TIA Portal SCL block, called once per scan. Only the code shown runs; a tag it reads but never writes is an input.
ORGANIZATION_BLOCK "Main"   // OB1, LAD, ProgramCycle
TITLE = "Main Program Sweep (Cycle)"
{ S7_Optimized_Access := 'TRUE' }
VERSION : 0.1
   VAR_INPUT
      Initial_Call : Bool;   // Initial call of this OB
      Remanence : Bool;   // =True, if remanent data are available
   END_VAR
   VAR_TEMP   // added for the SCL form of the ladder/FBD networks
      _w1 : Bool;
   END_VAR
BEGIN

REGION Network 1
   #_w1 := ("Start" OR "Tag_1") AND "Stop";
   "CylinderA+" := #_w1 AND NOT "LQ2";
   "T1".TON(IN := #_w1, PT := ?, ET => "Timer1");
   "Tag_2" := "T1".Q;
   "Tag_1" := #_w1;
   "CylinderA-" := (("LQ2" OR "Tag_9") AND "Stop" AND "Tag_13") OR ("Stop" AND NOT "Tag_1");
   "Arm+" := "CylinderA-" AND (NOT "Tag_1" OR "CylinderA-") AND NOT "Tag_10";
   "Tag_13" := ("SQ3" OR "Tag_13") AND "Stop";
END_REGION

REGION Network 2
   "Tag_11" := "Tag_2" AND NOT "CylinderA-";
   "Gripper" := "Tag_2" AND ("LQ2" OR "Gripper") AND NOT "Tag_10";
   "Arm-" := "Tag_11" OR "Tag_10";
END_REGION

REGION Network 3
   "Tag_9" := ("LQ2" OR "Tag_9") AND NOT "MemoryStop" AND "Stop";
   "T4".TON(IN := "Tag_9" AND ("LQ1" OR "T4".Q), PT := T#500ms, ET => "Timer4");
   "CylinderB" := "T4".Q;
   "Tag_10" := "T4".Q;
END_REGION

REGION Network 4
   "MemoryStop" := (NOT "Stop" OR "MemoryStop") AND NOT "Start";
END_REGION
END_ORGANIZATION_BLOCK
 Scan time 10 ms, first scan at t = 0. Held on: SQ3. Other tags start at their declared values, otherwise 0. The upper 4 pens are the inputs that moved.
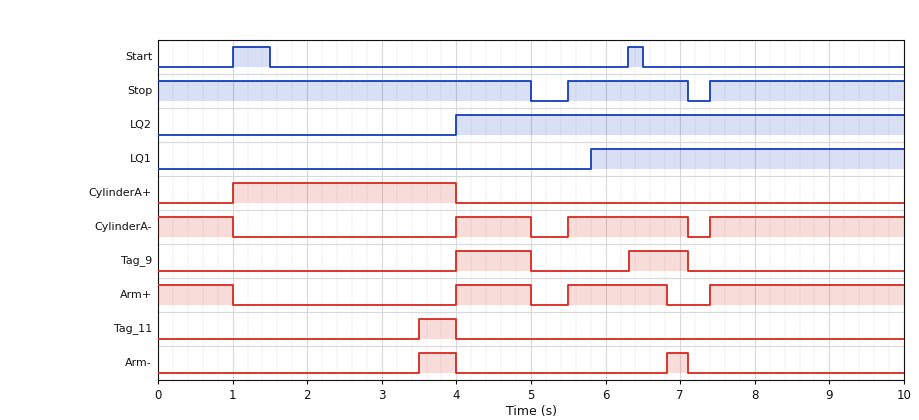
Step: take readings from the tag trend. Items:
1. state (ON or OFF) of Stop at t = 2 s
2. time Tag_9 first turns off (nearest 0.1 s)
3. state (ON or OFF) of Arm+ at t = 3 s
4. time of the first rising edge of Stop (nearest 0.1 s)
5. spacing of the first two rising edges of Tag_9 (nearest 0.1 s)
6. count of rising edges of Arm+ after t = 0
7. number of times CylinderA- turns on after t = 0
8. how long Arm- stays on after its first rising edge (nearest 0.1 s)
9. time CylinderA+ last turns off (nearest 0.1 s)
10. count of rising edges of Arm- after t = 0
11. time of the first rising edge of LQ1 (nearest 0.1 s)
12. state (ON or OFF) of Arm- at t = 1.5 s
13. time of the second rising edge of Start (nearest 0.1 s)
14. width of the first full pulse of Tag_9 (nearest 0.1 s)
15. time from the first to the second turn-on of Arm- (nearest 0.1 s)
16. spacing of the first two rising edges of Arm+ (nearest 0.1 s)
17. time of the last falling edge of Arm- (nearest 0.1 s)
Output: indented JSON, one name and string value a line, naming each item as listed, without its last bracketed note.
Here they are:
{
  "state (ON or OFF) of Stop at t = 2 s": "ON",
  "time Tag_9 first turns off": "5.0 s",
  "state (ON or OFF) of Arm+ at t = 3 s": "OFF",
  "time of the first rising edge of Stop": "5.5 s",
  "spacing of the first two rising edges of Tag_9": "2.3 s",
  "count of rising edges of Arm+ after t = 0": "3",
  "number of times CylinderA- turns on after t = 0": "3",
  "how long Arm- stays on after its first rising edge": "0.5 s",
  "time CylinderA+ last turns off": "4.0 s",
  "count of rising edges of Arm- after t = 0": "2",
  "time of the first rising edge of LQ1": "5.8 s",
  "state (ON or OFF) of Arm- at t = 1.5 s": "OFF",
  "time of the second rising edge of Start": "6.3 s",
  "width of the first full pulse of Tag_9": "1.0 s",
  "time from the first to the second turn-on of Arm-": "3.3 s",
  "spacing of the first two rising edges of Arm+": "1.5 s",
  "time of the last falling edge of Arm-": "7.1 s"
}
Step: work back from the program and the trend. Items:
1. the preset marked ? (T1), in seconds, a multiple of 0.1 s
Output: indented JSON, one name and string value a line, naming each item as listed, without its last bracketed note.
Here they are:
{
  "the preset marked ? (T1), in seconds, a multiple of 0.1 s": "2.5 s"
}
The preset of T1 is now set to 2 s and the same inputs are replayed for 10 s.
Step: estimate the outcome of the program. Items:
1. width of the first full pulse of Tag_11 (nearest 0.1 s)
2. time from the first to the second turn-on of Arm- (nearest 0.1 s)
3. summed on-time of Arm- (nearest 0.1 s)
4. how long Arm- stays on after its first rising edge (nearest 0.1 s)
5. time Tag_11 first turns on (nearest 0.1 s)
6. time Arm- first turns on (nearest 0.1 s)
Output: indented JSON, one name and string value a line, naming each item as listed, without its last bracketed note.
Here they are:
{
  "width of the first full pulse of Tag_11": "1.0 s",
  "time from the first to the second turn-on of Arm-": "3.8 s",
  "summed on-time of Arm-": "1.3 s",
  "how long Arm- stays on after its first rising edge": "1.0 s",
  "time Tag_11 first turns on": "3.0 s",
  "time Arm- first turns on": "3.0 s"
}
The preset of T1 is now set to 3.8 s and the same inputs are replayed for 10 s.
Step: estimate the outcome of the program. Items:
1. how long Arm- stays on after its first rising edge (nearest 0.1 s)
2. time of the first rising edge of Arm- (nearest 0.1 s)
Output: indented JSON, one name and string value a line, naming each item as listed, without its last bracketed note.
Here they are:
{
  "how long Arm- stays on after its first rising edge": "0.3 s",
  "time of the first rising edge of Arm-": "6.8 s"
}
